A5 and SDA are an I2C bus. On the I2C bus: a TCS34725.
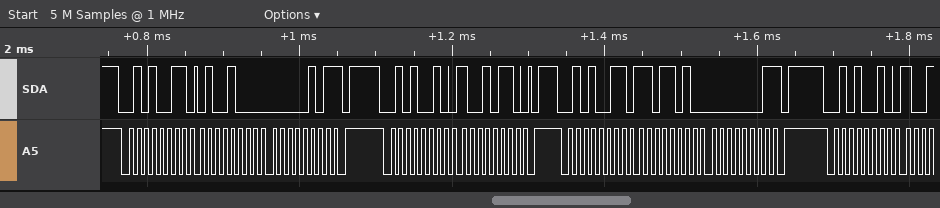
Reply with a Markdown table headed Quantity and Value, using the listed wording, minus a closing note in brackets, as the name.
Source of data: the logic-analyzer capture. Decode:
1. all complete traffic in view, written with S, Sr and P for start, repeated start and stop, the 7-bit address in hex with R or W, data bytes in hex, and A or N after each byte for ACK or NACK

| Quantity | Value |
|---|---|
| all complete traffic in view, written with S, Sr and P for start, repeated start and stop, the 7-bit address in hex with R or W, data bytes in hex, and A or N after each byte for ACK or NACK | S 29R A 48 A 05 N P S 29W A 96 A P S 29R A DA A 01 N P S 29W A |
